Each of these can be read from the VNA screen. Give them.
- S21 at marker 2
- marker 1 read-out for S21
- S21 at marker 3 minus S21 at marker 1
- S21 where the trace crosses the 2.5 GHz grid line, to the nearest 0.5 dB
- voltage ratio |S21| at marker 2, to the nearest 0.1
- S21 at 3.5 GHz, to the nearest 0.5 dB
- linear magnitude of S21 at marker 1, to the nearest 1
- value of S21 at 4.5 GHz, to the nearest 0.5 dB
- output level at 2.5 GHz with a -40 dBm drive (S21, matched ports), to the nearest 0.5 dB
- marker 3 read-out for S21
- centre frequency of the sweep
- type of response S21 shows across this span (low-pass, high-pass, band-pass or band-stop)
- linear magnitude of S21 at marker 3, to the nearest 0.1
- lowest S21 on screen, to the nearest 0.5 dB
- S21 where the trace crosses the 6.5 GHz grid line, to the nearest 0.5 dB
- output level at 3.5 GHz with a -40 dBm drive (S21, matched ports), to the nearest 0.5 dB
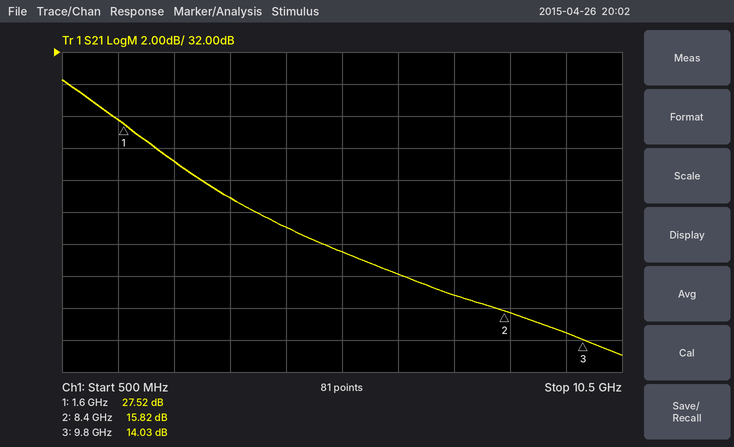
15.82 dB
27.52 dB
-13.49 dB
25.0 dB
6.2
23.0 dB
24
21.0 dB
-15.0 dBm
14.03 dB
5.5 GHz
low-pass
5.0
13.0 dB
18.0 dB
-17.0 dBm
